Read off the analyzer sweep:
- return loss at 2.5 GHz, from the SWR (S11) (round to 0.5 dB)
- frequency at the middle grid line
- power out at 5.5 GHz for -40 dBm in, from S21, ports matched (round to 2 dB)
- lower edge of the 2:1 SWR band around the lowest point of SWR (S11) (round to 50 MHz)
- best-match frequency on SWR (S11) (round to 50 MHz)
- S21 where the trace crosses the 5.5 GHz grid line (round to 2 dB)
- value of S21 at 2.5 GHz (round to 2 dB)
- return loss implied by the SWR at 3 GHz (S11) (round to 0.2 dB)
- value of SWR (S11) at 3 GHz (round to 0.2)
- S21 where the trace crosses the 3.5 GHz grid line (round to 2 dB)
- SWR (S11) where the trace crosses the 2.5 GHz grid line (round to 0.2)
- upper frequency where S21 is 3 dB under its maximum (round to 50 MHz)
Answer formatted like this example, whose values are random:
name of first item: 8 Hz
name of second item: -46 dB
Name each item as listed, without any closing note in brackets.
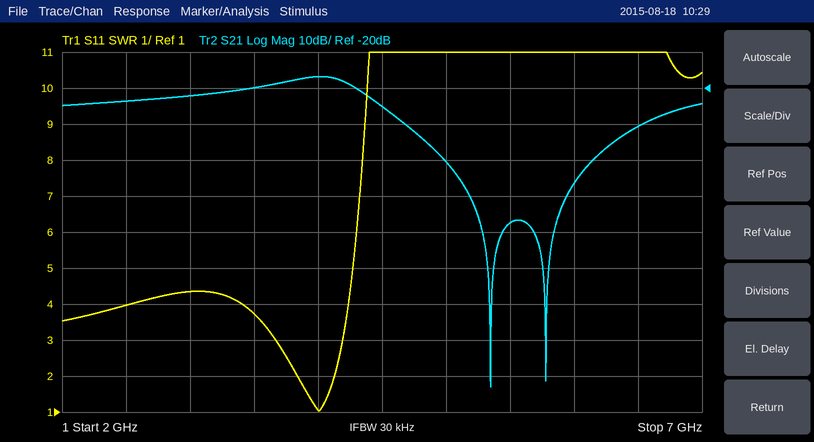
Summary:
return loss at 2.5 GHz, from the SWR (S11): 4.5 dB
frequency at the middle grid line: 4.5 GHz
power out at 5.5 GHz for -40 dBm in, from S21, ports matched: -98 dBm
lower edge of the 2:1 SWR band around the lowest point of SWR (S11): 3.85 GHz
best-match frequency on SWR (S11): 4.00 GHz
S21 where the trace crosses the 5.5 GHz grid line: -58 dB
value of S21 at 2.5 GHz: -24 dB
return loss implied by the SWR at 3 GHz (S11): 4.0 dB
value of SWR (S11) at 3 GHz: 4.4
S21 where the trace crosses the 3.5 GHz grid line: -20 dB
SWR (S11) where the trace crosses the 2.5 GHz grid line: 4.0
upper frequency where S21 is 3 dB under its maximum: 4.30 GHz
